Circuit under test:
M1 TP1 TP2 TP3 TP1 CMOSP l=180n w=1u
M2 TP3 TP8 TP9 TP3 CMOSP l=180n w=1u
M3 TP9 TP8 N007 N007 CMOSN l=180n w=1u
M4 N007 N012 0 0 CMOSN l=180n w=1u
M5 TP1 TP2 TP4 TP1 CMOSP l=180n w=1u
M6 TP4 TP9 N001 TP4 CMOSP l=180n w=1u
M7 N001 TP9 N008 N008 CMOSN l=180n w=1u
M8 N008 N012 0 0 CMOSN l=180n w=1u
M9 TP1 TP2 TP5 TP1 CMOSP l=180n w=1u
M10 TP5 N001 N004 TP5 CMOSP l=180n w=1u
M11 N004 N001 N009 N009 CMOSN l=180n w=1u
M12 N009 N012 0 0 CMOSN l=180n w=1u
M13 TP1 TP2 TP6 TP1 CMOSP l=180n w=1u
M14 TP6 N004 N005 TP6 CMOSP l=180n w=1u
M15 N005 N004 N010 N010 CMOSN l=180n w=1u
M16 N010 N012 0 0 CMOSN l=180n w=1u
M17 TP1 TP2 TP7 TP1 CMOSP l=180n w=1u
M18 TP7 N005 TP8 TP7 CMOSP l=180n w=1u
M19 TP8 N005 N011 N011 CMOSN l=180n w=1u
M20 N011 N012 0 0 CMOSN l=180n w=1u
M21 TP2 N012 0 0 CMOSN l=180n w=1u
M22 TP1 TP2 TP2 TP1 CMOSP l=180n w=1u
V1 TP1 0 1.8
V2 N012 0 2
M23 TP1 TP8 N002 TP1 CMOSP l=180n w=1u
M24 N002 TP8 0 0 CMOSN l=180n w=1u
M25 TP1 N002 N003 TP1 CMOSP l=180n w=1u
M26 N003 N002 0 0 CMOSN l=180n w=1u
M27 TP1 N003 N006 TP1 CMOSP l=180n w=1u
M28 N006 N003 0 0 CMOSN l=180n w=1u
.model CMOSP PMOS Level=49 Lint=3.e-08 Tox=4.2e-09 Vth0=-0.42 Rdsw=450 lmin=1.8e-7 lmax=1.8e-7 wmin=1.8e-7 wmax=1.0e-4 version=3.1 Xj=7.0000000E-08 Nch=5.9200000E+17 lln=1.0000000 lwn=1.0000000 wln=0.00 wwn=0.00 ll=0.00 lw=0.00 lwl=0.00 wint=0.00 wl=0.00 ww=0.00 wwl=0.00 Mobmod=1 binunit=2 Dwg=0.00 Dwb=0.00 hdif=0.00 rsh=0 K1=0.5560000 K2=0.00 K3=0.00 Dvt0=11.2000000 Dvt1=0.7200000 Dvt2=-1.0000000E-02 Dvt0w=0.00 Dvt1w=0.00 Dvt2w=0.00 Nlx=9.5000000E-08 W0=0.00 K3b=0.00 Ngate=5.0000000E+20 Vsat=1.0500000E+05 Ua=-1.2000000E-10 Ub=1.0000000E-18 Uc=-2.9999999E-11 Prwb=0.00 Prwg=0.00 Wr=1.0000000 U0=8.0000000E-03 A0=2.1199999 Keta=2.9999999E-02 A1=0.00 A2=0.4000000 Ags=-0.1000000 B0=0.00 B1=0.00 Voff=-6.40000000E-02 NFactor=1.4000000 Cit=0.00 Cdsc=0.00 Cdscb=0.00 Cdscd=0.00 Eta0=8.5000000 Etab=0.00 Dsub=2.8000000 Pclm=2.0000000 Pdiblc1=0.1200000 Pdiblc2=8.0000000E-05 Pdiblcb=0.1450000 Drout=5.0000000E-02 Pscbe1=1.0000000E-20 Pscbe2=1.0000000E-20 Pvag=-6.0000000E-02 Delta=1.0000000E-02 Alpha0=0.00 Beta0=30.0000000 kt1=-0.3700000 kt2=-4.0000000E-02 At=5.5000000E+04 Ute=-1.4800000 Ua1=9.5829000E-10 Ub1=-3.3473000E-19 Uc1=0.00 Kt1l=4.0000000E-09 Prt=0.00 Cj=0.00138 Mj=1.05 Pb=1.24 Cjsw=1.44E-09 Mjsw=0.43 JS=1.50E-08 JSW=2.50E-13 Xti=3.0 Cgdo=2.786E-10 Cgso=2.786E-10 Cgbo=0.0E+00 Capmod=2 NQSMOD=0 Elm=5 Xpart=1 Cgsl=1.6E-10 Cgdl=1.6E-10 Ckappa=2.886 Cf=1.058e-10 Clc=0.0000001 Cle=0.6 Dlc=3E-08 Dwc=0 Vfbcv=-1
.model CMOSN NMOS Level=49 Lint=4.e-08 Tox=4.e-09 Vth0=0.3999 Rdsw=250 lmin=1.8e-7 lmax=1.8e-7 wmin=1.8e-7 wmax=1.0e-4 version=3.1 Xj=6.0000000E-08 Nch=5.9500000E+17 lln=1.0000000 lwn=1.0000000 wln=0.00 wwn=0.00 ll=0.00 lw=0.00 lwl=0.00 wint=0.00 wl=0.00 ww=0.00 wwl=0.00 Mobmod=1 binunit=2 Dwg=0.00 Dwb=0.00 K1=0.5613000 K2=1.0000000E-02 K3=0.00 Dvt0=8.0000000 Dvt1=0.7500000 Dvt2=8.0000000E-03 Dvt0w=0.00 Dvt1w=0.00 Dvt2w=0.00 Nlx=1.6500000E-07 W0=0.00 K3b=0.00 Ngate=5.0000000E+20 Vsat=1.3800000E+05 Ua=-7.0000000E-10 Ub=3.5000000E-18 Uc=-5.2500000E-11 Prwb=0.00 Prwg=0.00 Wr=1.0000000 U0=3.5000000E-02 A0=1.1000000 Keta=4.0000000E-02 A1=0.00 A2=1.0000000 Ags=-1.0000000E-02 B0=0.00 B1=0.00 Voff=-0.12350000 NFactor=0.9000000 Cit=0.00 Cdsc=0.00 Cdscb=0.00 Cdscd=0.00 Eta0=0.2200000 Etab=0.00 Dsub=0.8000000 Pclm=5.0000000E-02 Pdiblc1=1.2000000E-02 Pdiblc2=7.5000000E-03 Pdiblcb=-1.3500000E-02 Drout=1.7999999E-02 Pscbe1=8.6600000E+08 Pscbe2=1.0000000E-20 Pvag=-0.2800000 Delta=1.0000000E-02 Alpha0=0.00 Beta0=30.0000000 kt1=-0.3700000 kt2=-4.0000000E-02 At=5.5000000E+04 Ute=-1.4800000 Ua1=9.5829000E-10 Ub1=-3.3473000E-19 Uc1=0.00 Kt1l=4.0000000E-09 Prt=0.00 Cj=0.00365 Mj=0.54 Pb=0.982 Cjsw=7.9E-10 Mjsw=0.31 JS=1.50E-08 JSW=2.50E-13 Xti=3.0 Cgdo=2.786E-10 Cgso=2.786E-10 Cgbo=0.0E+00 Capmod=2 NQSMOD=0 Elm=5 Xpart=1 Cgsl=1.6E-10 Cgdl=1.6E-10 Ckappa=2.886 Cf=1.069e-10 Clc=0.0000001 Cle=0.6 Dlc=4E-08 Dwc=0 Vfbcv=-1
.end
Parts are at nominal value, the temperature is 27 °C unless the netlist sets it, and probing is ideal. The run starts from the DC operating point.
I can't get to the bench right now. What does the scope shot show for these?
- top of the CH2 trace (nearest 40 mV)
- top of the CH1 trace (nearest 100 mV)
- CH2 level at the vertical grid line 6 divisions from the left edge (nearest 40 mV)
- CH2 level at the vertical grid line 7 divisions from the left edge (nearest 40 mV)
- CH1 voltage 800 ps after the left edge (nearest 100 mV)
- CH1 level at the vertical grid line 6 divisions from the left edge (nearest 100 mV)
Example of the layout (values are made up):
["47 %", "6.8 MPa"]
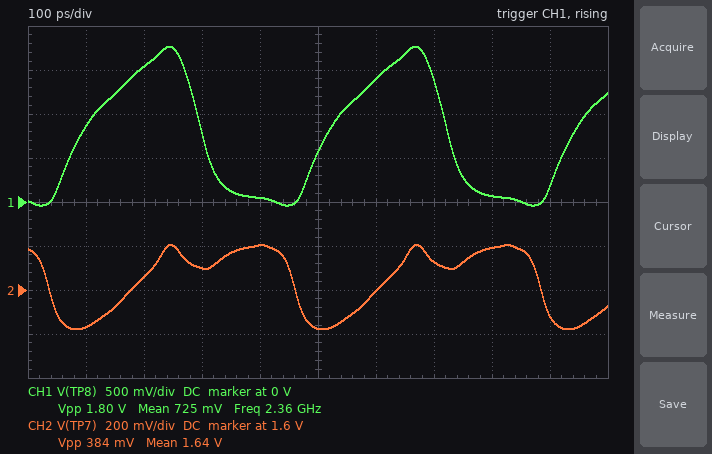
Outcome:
["1.80 V", "1.8 V", "1.60 V", "1.72 V", "100 mV", "1.4 V"]
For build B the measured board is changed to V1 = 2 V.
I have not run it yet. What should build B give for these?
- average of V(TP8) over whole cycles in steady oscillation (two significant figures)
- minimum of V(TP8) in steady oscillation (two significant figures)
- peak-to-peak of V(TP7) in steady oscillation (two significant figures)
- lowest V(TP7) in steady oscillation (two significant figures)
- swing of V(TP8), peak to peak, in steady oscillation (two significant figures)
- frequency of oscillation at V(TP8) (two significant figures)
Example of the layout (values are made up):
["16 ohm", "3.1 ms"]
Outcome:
["840 mV", "-40 mV", "430 mV", "1.6 V", "2.0 V", "2.6 GHz"]
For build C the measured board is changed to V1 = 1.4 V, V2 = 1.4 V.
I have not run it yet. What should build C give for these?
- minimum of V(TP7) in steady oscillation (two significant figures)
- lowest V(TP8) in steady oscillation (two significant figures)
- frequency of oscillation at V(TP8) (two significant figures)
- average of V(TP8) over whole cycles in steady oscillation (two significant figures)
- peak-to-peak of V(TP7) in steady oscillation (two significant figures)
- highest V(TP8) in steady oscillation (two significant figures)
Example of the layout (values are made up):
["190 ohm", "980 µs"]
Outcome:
["1.1 V", "-41 mV", "1.8 GHz", "600 mV", "300 mV", "1.4 V"]
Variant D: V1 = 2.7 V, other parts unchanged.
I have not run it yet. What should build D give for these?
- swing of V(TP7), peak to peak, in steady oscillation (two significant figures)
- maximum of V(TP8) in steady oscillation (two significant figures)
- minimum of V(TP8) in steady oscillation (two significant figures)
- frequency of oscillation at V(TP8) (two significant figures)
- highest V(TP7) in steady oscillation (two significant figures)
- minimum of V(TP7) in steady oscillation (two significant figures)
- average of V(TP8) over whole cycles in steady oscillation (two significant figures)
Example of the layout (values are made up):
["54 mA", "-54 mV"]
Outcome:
["610 mV", "2.6 V", "-30 mV", "3.0 GHz", "2.7 V", "2.1 V", "1.1 V"]
